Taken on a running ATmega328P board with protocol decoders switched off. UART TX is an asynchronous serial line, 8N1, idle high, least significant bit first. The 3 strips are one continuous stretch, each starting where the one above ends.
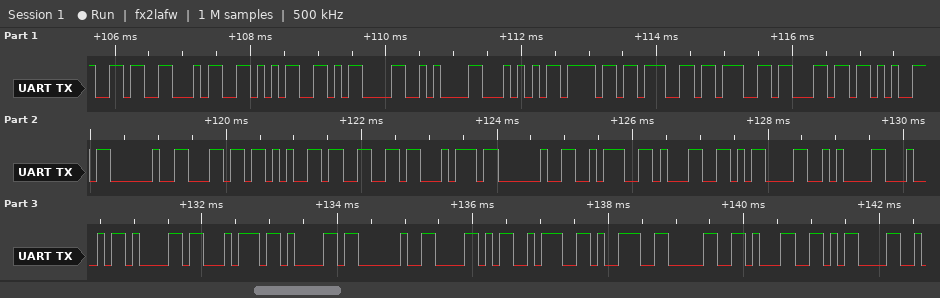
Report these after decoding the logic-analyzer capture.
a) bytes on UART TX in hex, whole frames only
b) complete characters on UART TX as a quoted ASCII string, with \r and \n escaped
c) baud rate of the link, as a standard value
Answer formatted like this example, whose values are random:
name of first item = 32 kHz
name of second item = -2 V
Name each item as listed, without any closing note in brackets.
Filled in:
bytes on UART TX in hex, whole frames only = 0x36 0x34 0x35 0x0D 0x0A 0x54 0x6F 0x67 0x67 0x6C 0x65 0x20 0x6C 0x65 0x66 0x74 0x20 0x3A 0x31 0x0D 0x0A 0x44 0x61 0x74 0x61 0x20 0x58 0x3A 0x39 0x30 0x31 0x0D
complete characters on UART TX as a quoted ASCII string, with \r and \n escaped = "645\r\nToggle left :1\r\nData X:901\r"
baud rate of the link, as a standard value = 9600 baud
